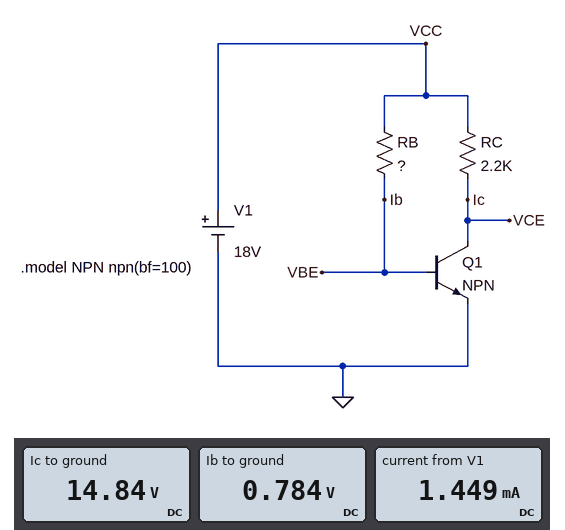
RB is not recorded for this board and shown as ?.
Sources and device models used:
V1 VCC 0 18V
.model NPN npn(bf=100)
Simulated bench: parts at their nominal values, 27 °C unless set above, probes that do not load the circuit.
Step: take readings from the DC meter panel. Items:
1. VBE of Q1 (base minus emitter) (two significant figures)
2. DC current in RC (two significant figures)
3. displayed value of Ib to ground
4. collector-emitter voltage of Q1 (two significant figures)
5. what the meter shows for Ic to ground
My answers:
780 mV
1.4 mA
0.784 V
15 V
14.84 V
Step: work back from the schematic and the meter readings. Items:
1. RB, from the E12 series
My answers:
1.2 MΩ
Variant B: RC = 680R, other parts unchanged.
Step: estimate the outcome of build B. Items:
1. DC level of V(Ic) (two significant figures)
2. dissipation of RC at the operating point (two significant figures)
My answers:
17 V
1.4 mW
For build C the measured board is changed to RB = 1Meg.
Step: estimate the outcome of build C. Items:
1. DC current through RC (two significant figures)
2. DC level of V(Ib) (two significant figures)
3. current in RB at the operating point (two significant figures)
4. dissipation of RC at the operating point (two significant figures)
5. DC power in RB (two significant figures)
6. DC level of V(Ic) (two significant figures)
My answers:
1.7 mA
790 mV
17 µA
6.5 mW
300 µW
14 V
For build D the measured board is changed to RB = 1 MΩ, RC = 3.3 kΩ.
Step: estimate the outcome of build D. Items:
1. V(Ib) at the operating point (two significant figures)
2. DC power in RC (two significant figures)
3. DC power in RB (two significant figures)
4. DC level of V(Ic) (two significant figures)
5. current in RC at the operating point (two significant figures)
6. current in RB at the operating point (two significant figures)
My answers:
790 mV
9.8 mW
300 µW
12 V
1.7 mA
17 µA
